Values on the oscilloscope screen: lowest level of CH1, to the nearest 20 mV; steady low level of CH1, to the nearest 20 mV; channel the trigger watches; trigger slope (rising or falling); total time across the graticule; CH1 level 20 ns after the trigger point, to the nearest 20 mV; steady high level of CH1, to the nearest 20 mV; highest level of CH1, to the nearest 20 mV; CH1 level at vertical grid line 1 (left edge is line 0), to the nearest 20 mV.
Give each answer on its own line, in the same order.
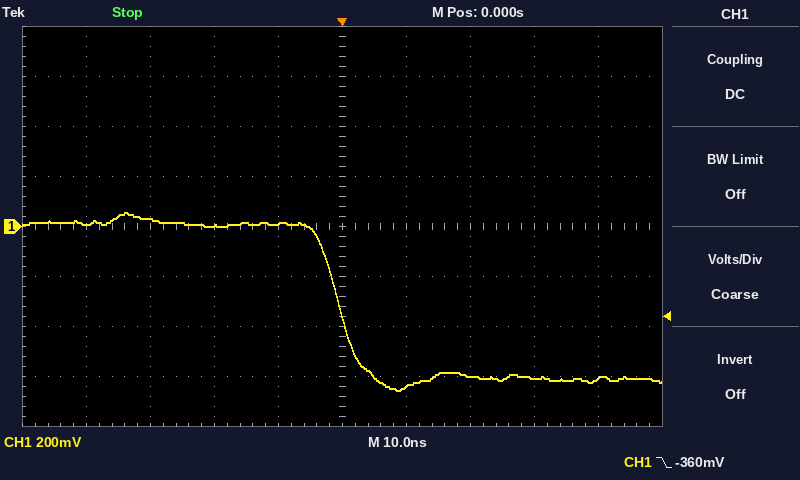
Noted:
-660 mV
-600 mV
CH1
falling
100 ns
-600 mV
20 mV
60 mV
0 mV
